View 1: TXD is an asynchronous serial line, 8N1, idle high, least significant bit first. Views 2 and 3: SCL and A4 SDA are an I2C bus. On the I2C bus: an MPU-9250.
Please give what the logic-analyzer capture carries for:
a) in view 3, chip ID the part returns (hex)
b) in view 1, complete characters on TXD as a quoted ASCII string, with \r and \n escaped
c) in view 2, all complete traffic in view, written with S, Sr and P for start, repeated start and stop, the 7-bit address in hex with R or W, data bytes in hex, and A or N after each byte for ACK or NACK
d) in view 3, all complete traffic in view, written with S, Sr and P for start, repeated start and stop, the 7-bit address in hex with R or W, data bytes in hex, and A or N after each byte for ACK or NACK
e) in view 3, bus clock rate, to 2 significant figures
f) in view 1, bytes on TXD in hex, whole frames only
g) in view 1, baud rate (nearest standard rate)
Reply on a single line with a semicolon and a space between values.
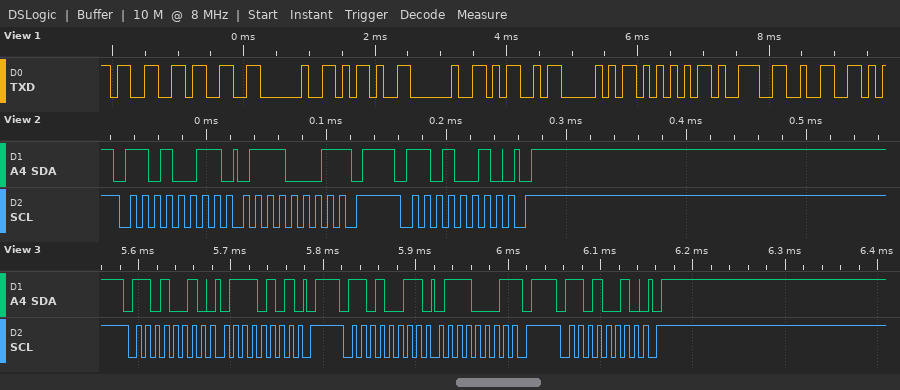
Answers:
0x71; "33 - MPU92"; S 69R A 71 N P S 69W A P; S 69W A 75 A P S 69R A 71 N P S 69W A P; 100 kHz; 0x33 0x33 0x20 0x2D 0x20 0x4D 0x50 0x55 0x39 0x32; 9600 baud
